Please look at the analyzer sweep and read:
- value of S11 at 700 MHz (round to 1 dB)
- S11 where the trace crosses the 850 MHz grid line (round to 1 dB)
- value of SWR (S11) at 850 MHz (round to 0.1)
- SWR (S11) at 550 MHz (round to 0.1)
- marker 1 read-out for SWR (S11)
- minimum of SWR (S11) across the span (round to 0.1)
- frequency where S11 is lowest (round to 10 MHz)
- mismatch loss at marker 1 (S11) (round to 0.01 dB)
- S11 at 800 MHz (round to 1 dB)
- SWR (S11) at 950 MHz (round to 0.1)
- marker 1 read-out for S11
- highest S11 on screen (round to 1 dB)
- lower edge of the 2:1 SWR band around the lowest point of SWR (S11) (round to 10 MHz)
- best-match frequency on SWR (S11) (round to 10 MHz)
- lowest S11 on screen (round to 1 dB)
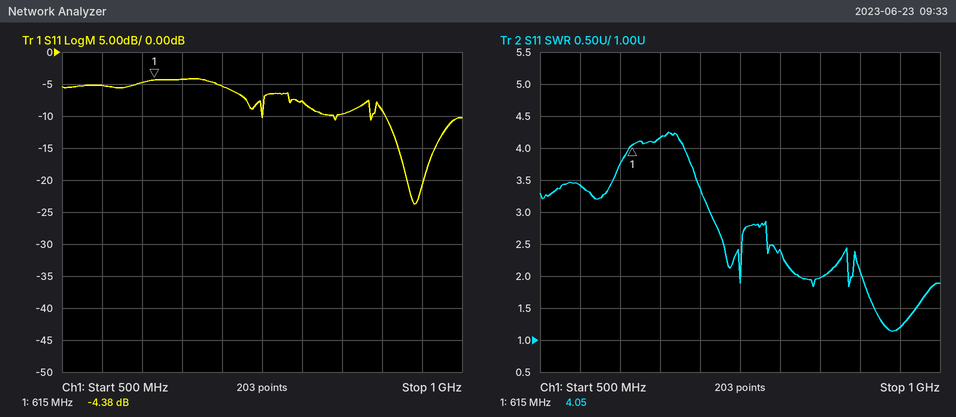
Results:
-5 dB
-10 dB
2.0
3.4
4.05
1.1
940 MHz
1.97 dB
-8 dB
1.2
-4.38 dB
-4 dB
900 MHz
940 MHz
-24 dB
